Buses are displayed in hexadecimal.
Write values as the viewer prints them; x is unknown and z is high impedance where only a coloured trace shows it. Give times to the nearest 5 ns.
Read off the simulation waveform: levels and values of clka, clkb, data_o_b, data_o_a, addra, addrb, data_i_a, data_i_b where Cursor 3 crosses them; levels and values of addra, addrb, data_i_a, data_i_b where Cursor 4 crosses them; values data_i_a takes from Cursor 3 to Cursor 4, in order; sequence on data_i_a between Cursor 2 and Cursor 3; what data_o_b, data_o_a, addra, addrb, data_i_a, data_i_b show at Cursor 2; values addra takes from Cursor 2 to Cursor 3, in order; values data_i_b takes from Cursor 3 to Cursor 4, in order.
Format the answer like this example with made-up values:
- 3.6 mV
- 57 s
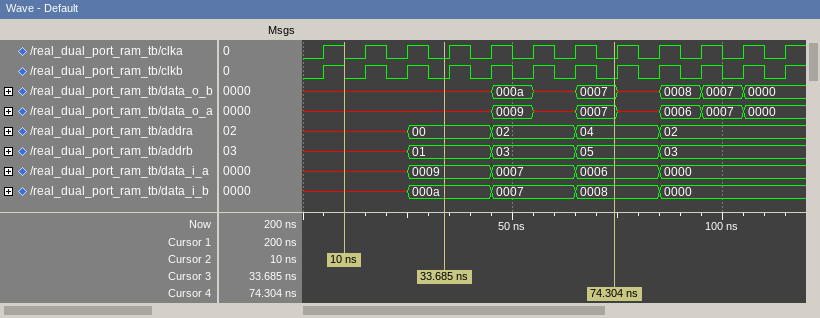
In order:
- clka=0, clkb=0, data_o_b=x, data_o_a=x, addra=00, addrb=01, data_i_a=0009, data_i_b=000a
- addra=04, addrb=05, data_i_a=0006, data_i_b=0008
- 0009, 0007, 0006
- x, 0009
- data_o_b=x, data_o_a=x, addra=x, addrb=x, data_i_a=x, data_i_b=x
- x, 00
- 000a, 0007, 0008
